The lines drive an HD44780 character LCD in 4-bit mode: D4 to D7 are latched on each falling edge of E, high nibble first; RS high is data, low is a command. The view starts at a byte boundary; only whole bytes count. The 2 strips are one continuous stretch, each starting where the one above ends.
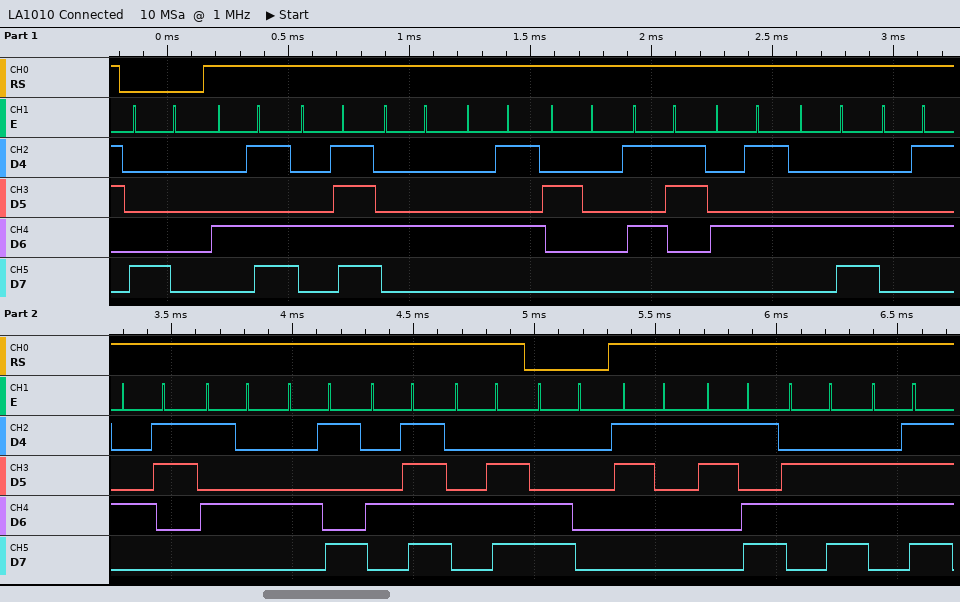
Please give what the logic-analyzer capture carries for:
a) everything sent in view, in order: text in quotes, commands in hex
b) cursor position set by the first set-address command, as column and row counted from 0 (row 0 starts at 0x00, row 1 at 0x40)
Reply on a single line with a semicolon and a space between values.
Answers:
0x80 "MODE SELECTION" 0xC0 "1=no"; column 0, row 0
